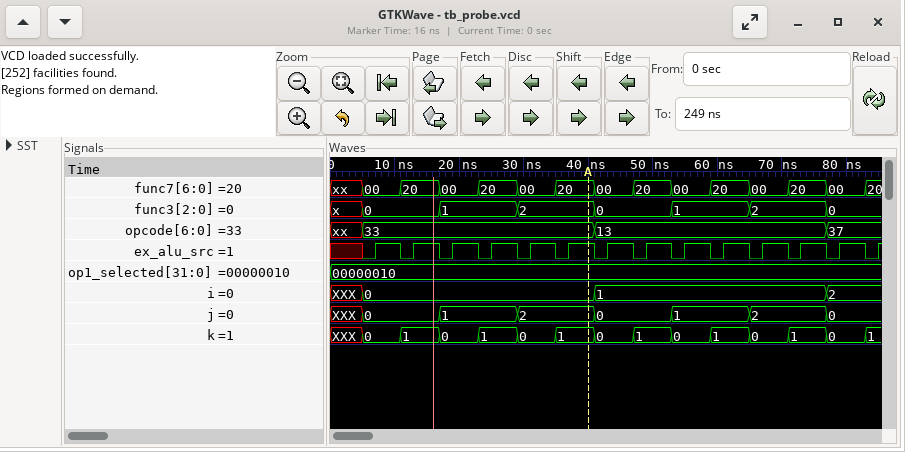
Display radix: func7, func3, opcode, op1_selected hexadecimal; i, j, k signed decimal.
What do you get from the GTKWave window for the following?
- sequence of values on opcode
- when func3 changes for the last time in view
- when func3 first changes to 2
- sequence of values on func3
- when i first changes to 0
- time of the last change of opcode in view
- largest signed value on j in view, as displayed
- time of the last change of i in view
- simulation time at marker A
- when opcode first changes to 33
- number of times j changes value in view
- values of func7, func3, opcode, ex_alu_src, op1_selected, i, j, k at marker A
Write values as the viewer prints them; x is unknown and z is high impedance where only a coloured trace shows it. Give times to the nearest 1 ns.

xx, 33, 13, 37
77 ns
29 ns
x, 0, 1, 2, 0, 1, 2, 0
5 ns
77 ns
2
77 ns
40 ns
5 ns
7
func7=20, func3=2, opcode=33, ex_alu_src=1, op1_selected=00000010, i=0, j=2, k=1
